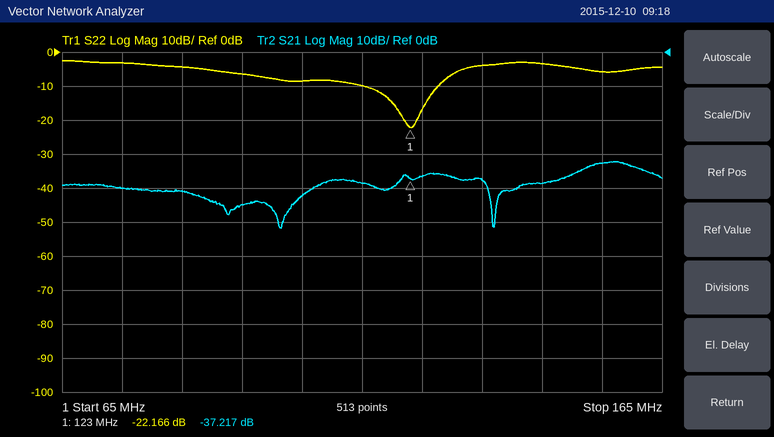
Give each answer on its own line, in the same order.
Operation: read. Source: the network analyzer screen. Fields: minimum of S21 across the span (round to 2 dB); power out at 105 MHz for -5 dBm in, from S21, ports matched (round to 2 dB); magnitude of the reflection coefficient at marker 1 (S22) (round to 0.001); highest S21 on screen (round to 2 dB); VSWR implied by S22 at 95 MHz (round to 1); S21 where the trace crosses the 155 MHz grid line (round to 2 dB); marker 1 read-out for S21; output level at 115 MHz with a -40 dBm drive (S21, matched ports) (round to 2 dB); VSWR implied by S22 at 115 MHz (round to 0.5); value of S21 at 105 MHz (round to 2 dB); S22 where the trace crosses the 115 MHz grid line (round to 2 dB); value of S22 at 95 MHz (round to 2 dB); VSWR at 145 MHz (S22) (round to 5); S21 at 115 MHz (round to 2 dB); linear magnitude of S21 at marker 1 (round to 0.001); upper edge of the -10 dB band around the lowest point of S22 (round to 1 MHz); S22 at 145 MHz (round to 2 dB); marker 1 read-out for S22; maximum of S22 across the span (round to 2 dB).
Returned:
-52 dB
-48 dBm
0.078
-32 dB
3
-32 dB
-37.217 dB
-78 dBm
2.0
-42 dB
-10 dB
-6 dB
5
-38 dB
0.014
128 MHz
-4 dB
-22.166 dB
-2 dB
